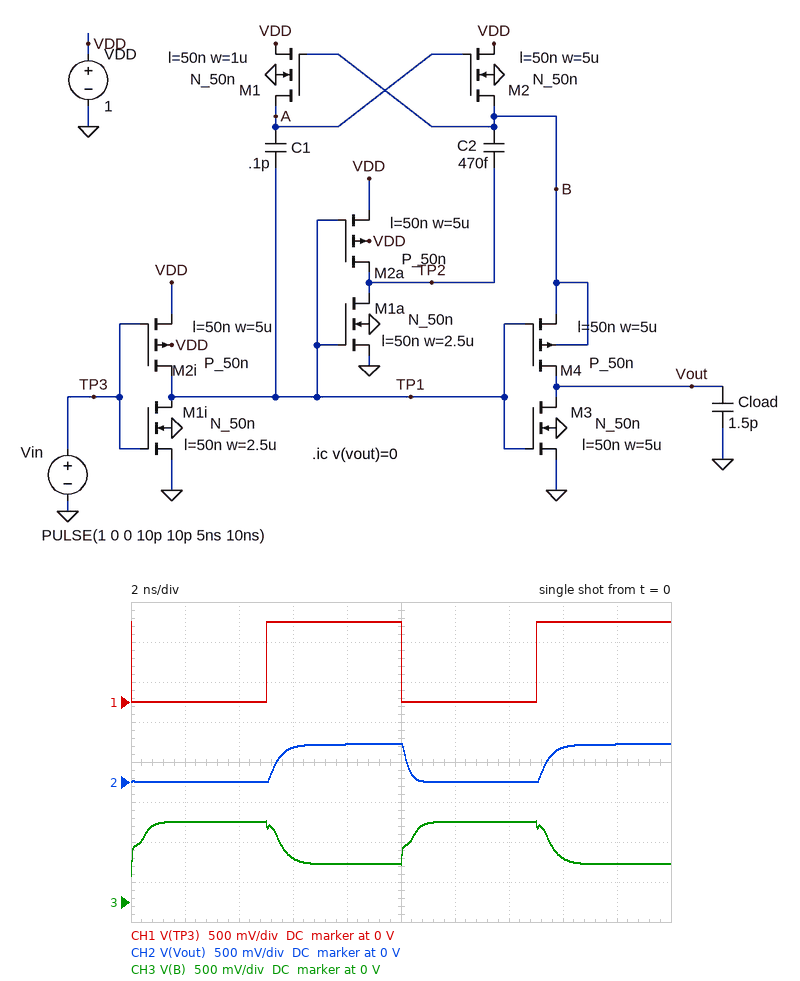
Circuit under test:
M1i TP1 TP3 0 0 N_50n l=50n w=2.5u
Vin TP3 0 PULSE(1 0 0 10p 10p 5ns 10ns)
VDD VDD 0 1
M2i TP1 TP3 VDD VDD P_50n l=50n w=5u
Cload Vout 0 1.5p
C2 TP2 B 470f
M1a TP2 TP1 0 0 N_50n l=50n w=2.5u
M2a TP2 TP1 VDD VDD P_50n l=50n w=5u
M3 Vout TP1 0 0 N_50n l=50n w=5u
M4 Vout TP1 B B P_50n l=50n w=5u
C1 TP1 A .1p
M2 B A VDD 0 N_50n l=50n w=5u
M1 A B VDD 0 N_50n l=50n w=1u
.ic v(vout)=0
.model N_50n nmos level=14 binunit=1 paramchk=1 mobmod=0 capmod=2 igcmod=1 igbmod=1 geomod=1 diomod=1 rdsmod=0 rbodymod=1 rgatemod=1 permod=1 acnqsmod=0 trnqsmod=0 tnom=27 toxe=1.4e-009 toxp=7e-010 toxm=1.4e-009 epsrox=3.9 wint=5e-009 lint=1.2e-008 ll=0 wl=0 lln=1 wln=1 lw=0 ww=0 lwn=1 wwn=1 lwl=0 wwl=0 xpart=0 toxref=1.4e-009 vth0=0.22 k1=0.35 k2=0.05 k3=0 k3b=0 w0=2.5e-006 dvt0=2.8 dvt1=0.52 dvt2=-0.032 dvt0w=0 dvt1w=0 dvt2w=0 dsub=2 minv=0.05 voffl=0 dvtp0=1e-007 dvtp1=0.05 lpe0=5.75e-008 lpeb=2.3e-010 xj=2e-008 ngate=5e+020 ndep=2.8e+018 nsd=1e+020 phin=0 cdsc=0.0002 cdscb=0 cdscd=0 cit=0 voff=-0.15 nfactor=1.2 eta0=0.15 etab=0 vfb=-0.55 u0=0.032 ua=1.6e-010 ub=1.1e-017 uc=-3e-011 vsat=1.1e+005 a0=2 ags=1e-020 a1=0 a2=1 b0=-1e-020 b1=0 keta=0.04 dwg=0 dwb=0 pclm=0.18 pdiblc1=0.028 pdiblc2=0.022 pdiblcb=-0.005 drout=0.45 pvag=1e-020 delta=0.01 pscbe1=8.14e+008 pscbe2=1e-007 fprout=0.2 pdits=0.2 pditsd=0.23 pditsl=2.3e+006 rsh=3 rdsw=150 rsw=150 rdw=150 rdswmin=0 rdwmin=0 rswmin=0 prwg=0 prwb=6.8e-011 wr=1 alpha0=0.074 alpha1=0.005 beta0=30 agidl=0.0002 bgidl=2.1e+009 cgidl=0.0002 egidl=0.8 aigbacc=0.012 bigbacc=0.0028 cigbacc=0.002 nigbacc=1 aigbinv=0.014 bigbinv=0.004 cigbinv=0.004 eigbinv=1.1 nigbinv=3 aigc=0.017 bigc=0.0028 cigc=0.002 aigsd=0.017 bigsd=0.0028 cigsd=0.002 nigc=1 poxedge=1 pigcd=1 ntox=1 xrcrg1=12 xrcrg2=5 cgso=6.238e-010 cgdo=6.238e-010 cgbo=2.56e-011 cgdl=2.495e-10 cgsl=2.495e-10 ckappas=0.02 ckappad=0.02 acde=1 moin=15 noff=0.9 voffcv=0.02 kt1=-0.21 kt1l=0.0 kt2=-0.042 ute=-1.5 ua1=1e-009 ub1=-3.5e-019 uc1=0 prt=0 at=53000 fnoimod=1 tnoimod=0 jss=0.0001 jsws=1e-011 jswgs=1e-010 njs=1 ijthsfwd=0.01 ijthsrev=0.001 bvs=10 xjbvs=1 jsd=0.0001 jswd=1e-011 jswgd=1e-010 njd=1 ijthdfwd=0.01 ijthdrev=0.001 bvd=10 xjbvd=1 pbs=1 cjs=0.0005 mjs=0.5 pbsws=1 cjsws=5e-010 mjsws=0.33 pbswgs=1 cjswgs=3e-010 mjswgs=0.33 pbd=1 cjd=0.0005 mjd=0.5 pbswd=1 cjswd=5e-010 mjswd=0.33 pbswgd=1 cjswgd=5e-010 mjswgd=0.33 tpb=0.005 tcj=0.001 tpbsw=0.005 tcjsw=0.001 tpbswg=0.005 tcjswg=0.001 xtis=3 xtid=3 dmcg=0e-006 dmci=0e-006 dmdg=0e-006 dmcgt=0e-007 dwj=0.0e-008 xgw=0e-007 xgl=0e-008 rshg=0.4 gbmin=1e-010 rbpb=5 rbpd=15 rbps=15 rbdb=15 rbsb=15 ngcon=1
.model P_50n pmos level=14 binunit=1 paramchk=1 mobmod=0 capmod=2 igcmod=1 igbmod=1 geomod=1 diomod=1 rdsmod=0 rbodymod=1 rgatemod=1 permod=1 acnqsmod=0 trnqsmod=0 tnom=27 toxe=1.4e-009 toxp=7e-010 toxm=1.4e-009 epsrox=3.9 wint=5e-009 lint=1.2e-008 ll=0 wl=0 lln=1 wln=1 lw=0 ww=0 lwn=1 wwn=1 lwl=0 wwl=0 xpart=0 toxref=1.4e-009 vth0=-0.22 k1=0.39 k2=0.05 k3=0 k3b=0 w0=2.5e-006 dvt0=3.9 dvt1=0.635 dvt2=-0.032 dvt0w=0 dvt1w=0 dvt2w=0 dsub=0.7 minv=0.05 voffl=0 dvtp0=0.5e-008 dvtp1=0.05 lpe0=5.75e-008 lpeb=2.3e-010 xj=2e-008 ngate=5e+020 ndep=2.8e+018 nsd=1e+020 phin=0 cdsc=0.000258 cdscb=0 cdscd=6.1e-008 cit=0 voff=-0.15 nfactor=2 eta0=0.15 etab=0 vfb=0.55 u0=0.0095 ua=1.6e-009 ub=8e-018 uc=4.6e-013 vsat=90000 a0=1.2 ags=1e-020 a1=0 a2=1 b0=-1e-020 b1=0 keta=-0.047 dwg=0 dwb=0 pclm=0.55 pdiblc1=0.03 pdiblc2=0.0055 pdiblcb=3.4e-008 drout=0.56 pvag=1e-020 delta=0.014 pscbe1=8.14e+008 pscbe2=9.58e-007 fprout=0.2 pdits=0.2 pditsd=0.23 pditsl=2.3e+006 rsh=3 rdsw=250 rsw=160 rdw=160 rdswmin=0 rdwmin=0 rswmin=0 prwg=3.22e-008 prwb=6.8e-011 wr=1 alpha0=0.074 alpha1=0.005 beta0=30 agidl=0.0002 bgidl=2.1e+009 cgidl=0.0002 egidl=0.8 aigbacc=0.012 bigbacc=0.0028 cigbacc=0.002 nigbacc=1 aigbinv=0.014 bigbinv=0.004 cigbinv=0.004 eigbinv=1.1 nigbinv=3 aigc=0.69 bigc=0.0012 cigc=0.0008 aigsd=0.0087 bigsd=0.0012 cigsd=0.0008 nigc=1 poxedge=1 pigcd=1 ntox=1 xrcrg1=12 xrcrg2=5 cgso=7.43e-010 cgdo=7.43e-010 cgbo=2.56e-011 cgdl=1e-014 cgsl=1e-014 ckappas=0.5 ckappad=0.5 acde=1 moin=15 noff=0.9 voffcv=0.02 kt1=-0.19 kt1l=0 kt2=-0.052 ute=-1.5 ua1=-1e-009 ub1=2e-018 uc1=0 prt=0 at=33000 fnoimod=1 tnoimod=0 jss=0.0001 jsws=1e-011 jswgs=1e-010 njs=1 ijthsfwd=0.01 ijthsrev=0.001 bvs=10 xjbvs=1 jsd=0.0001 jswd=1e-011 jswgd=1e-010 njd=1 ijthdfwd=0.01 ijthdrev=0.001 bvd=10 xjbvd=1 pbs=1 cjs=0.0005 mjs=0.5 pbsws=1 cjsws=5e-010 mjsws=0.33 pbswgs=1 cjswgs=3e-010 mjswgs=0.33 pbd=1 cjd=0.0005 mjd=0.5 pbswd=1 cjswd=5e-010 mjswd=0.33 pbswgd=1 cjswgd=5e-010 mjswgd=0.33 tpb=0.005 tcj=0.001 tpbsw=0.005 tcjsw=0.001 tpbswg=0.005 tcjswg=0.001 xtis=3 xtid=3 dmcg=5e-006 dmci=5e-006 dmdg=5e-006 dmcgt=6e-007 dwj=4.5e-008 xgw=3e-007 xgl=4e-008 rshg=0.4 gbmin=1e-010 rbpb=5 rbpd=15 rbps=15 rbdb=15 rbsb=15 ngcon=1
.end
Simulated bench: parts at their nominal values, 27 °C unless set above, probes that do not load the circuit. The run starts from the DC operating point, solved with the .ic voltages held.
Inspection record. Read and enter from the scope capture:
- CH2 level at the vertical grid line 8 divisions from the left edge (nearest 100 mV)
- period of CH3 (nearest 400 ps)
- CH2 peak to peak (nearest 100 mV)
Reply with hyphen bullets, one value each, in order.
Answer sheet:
- 400 mV
- 10.0 ns
- 500 mV
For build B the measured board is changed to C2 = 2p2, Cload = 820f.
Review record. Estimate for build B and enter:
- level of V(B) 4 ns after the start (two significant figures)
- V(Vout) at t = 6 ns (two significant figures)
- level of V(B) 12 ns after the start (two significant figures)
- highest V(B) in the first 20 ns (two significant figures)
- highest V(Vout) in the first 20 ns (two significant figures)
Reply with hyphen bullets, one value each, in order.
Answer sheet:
- 970 mV
- 1.2 V
- 980 mV
- 1.5 V
- 1.4 V
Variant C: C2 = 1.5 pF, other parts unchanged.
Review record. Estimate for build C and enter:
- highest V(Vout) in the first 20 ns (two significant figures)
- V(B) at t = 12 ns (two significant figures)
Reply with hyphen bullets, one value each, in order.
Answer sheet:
- 990 mV
- 970 mV
